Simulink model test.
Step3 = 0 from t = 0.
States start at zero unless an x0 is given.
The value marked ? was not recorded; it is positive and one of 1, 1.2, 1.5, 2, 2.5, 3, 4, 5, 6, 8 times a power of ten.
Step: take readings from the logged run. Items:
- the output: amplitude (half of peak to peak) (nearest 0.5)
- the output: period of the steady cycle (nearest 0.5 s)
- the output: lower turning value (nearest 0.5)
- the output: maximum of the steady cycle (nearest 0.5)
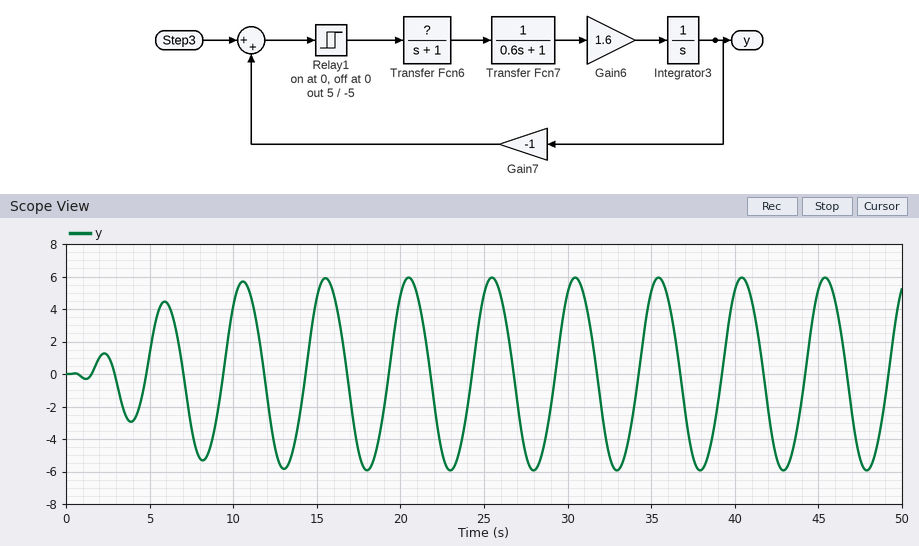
6.0
5.0 s
-6.0
6.0
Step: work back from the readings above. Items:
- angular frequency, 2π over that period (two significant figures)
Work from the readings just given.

1.3 rad/s
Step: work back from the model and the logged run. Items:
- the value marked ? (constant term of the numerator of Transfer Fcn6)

1.5
